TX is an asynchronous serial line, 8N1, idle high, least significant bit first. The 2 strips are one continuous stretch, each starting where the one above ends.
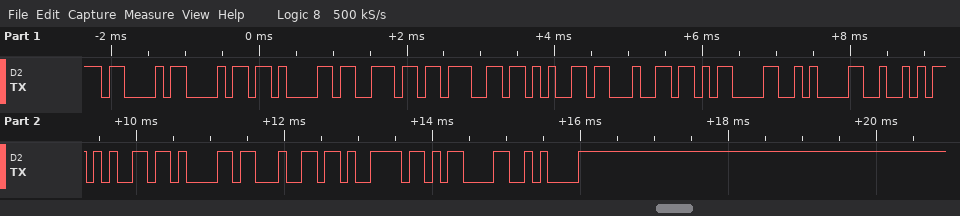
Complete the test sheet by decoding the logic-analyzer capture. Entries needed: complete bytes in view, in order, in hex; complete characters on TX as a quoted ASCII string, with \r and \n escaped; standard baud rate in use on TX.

43 68 61 6E 67 65 64 0D 0A 52 65 61 64 79 0D 0A
"Changed\r\nReady\r\n"
9600 baud
